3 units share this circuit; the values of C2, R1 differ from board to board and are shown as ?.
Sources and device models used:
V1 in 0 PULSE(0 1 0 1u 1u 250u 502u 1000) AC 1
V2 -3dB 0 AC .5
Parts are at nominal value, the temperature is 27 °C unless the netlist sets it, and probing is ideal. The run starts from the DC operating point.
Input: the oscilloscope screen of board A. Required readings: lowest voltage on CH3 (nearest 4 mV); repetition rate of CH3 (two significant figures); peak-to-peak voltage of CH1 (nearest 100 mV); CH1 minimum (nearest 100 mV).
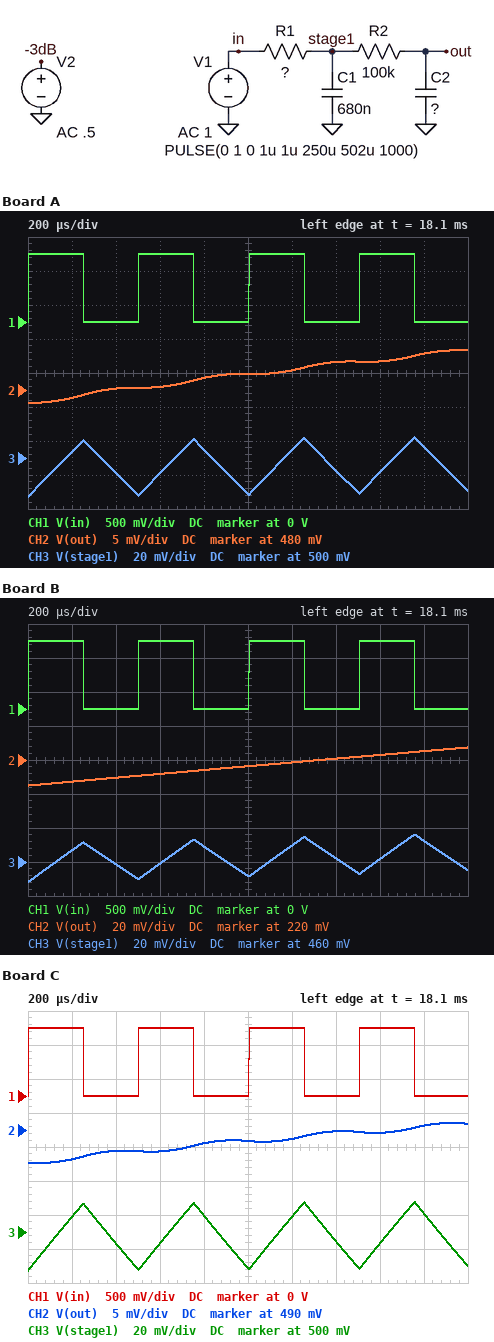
476 mV
2.0 kHz
1.0 V
0 V
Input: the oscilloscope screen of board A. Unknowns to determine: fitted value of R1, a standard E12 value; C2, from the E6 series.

5.6 kΩ
33 nF
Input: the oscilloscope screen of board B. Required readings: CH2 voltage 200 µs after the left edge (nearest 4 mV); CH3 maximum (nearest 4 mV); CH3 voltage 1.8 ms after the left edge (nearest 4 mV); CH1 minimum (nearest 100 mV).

208 mV
476 mV
472 mV
0 V
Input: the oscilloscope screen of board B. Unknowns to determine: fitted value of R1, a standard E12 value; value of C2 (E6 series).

8.2 kΩ
220 nF
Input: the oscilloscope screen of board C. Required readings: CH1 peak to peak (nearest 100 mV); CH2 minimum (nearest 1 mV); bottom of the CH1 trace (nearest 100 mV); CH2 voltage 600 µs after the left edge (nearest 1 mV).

1.0 V
485 mV
0 V
487 mV
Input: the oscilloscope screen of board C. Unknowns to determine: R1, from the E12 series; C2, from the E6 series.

4.7 kΩ
33 nF
